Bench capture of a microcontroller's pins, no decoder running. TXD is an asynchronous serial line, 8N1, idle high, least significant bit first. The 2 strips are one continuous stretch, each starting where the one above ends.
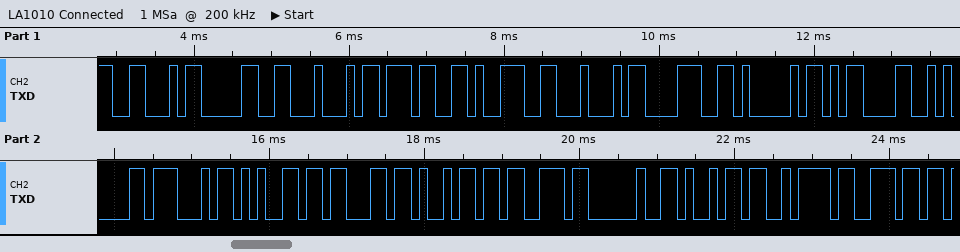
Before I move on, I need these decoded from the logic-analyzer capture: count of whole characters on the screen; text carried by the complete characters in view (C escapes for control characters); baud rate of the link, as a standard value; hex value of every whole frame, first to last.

19
"F0D79D8A\r\nGecis izn"
9600 baud
46 30 44 37 39 44 38 41 0D 0A 47 65 63 69 73 20 69 7A 6E
